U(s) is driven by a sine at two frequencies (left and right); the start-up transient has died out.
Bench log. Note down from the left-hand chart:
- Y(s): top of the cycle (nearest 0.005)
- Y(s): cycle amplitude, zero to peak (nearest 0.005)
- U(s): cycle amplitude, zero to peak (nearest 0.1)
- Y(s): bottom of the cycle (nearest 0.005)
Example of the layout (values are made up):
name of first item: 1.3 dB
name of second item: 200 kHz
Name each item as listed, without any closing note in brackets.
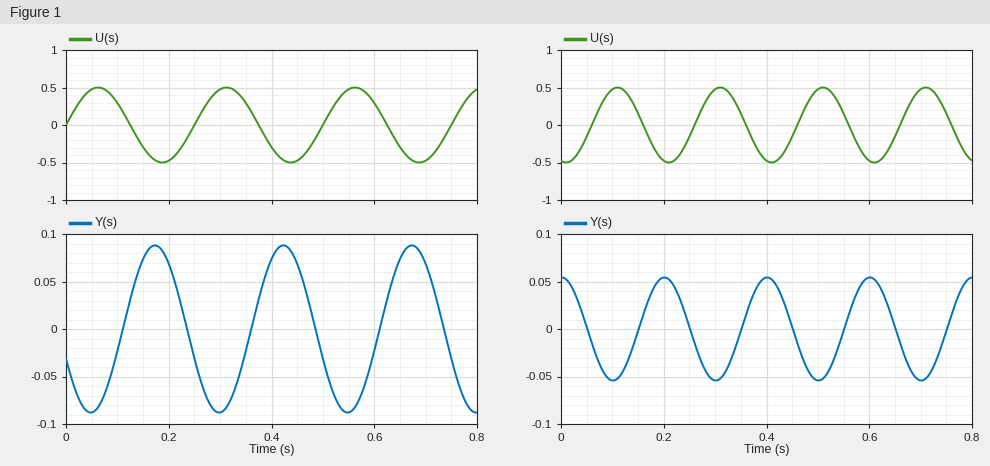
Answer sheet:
Y(s): top of the cycle: 0.090
Y(s): cycle amplitude, zero to peak: 0.090
U(s): cycle amplitude, zero to peak: 0.5
Y(s): bottom of the cycle: -0.090
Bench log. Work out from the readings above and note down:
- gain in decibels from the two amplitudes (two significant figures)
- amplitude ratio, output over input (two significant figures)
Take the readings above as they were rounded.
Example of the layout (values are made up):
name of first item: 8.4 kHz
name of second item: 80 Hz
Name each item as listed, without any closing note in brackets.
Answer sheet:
gain in decibels from the two amplitudes: -15 dB
amplitude ratio, output over input: 0.18
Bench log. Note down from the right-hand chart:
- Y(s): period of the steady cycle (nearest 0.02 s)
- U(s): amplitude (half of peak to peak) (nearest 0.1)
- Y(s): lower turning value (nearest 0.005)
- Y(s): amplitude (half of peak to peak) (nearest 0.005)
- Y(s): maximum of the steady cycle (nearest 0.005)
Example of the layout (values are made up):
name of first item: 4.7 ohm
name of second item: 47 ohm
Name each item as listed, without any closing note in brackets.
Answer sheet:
Y(s): period of the steady cycle: 0.20 s
U(s): amplitude (half of peak to peak): 0.5
Y(s): lower turning value: -0.055
Y(s): amplitude (half of peak to peak): 0.055
Y(s): maximum of the steady cycle: 0.055
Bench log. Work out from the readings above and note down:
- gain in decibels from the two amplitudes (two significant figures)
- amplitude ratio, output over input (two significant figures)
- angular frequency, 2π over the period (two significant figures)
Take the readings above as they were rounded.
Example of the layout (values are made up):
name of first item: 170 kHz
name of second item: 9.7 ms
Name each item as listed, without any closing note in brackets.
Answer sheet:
gain in decibels from the two amplitudes: -19 dB
amplitude ratio, output over input: 0.11
angular frequency, 2π over the period: 31 rad/s
